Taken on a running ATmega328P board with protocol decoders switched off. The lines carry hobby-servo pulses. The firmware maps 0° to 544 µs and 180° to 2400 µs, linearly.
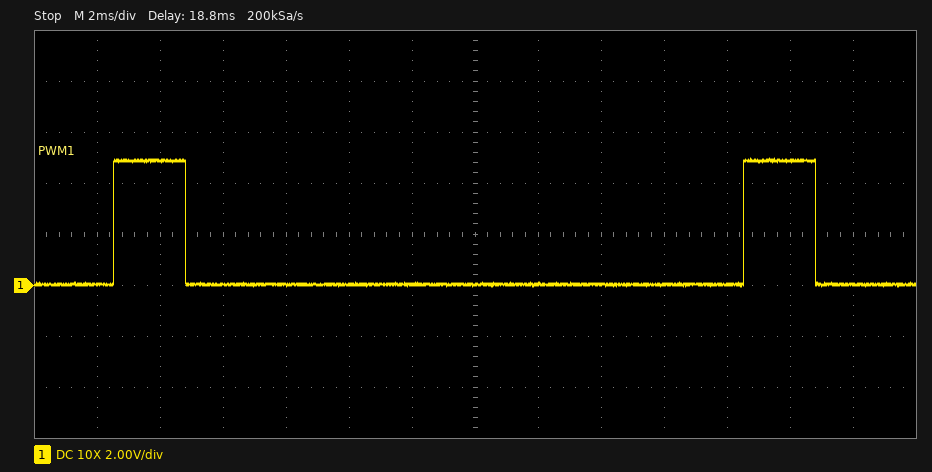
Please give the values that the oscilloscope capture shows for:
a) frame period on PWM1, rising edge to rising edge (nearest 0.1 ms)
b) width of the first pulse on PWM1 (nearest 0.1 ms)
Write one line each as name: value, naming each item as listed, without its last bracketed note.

frame period on PWM1, rising edge to rising edge: 20.0 ms
width of the first pulse on PWM1: 2.3 ms
